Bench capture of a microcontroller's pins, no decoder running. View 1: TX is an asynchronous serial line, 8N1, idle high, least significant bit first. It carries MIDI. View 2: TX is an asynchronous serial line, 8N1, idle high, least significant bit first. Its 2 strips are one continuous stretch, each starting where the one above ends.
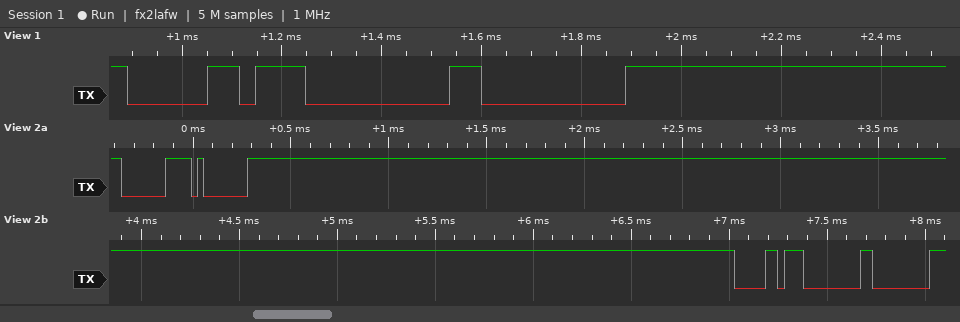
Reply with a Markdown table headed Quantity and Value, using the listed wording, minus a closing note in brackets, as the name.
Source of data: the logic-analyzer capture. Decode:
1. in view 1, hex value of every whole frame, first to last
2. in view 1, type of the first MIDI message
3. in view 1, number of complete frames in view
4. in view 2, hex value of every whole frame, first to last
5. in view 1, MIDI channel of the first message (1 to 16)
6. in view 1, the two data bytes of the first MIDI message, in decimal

| Quantity | Value |
|---|---|
| in view 1, hex value of every whole frame, first to last | B0 00 00 |
| in view 1, type of the first MIDI message | Control Change |
| in view 1, number of complete frames in view | 3 |
| in view 2, hex value of every whole frame, first to last | 0xC0 0x01 0xB0 0x00 0x00 |
| in view 1, MIDI channel of the first message | 1 |
| in view 1, the two data bytes of the first MIDI message, in decimal | 0, 0 |
